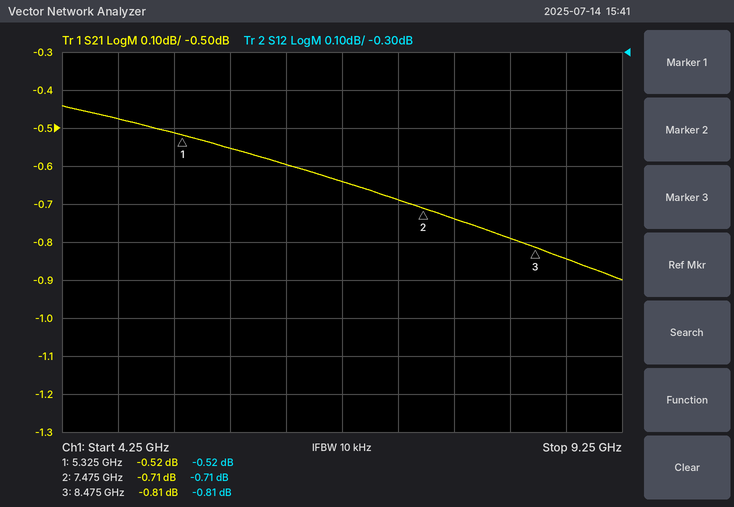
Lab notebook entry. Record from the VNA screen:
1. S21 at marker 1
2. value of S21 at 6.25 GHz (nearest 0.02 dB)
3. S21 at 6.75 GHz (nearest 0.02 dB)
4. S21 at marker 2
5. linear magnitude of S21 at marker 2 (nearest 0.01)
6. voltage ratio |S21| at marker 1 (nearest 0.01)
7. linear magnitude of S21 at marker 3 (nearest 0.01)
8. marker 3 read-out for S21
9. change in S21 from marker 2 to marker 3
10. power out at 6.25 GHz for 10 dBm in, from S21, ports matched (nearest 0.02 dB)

-0.52 dB
-0.60 dB
-0.64 dB
-0.71 dB
0.92
0.94
0.91
-0.81 dB
-0.10 dB
9.40 dBm
